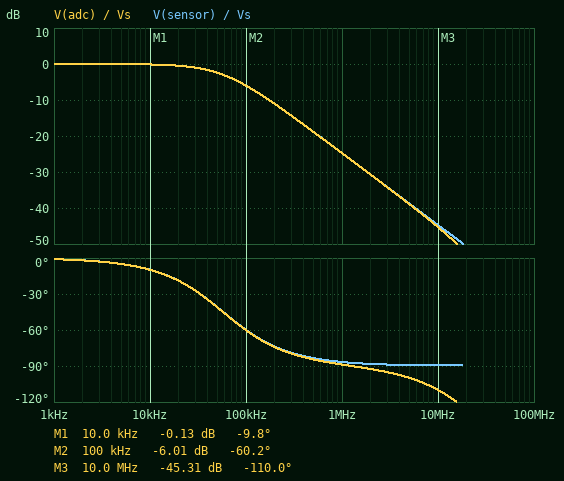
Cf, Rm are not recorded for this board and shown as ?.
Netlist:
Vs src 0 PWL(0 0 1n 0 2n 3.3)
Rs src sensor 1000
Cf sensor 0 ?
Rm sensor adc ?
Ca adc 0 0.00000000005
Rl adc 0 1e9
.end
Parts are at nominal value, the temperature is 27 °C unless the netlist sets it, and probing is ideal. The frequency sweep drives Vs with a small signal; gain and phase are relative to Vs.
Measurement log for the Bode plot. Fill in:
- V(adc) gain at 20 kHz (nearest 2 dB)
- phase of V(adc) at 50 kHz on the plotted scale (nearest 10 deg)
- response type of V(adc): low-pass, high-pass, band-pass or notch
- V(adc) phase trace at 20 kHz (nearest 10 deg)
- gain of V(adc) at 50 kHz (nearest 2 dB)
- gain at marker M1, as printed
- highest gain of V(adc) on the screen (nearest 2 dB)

0 dB
-40 deg
low-pass
-20 deg
-2 dB
-0.13 dB
0 dB
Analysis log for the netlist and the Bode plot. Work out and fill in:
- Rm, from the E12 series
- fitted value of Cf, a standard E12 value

120 Ω
2.7 nF
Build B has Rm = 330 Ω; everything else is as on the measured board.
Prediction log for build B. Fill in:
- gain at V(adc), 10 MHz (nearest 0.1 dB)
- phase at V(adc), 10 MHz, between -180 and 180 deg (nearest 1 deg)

-47.8 dB
-135 deg
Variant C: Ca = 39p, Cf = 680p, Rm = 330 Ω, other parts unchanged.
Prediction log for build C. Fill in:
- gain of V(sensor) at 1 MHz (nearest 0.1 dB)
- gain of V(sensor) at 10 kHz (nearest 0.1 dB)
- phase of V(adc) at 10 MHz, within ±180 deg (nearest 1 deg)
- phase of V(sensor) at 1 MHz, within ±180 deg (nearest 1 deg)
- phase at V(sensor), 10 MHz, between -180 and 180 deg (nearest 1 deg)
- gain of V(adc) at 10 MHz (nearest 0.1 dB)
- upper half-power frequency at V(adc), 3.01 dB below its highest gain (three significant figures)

-13.3 dB
0 dB
-126 deg
-77 deg
-87 deg
-35.1 dB
221 kHz
